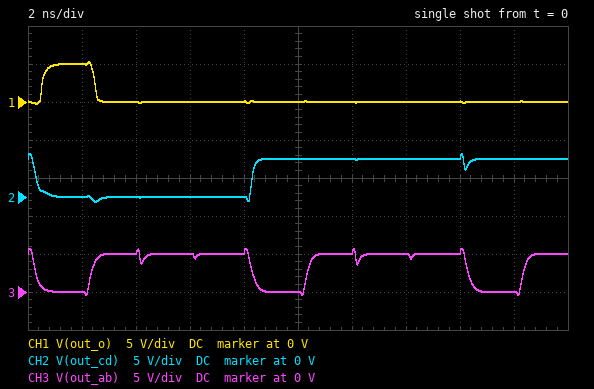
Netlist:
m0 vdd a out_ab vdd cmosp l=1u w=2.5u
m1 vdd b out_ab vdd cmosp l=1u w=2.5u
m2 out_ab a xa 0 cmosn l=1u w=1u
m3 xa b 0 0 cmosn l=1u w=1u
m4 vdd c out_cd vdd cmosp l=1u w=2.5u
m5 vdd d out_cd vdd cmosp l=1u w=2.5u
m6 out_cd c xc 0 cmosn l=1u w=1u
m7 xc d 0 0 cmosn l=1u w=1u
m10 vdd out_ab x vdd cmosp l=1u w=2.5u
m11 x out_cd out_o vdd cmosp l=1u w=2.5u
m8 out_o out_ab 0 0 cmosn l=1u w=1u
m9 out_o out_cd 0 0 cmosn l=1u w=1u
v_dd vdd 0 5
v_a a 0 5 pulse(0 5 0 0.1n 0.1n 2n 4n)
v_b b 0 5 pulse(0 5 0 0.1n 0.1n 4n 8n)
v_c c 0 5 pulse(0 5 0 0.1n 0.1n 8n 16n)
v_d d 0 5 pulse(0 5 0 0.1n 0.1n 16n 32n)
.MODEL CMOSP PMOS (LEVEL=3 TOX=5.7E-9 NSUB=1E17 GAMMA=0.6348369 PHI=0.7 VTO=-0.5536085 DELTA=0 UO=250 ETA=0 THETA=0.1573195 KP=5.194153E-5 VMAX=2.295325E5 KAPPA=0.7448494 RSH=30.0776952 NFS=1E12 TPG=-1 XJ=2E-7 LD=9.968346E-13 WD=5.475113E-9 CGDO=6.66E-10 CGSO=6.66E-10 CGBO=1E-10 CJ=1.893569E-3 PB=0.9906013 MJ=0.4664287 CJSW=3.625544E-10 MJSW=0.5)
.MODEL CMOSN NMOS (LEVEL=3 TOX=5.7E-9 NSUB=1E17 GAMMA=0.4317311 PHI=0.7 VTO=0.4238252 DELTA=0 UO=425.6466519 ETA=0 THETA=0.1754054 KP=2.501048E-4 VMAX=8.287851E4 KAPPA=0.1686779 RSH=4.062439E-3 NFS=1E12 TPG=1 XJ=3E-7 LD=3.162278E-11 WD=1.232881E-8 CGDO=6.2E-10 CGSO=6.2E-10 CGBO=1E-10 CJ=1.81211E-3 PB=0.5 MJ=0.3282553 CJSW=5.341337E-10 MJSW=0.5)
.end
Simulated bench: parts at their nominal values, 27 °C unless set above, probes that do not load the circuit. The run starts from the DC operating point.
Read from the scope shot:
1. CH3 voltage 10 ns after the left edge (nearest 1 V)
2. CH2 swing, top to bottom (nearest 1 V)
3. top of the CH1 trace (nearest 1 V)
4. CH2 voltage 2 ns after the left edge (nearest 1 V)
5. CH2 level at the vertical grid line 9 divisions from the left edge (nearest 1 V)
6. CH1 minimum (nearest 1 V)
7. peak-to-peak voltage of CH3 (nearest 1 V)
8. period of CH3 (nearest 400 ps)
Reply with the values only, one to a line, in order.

0 V
6 V
5 V
0 V
5 V
0 V
6 V
8.0 ns
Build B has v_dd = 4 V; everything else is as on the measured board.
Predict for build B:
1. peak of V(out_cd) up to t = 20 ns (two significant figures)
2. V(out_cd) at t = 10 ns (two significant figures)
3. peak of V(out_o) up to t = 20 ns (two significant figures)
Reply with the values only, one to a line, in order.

4.6 V
4.0 V
4.3 V
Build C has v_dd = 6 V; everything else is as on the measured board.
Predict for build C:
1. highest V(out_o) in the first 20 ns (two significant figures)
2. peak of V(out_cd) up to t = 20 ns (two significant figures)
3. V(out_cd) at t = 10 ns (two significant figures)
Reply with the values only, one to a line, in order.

6.3 V
6.6 V
6.0 V
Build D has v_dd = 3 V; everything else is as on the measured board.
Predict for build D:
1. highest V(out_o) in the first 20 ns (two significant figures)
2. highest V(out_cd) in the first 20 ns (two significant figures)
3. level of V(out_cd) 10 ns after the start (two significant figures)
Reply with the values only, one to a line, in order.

3.2 V
3.6 V
3.0 V
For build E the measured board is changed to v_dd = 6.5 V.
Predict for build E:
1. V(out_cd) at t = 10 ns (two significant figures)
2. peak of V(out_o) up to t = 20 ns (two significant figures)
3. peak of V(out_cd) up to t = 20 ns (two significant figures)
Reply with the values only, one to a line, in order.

6.5 V
6.8 V
7.1 V
